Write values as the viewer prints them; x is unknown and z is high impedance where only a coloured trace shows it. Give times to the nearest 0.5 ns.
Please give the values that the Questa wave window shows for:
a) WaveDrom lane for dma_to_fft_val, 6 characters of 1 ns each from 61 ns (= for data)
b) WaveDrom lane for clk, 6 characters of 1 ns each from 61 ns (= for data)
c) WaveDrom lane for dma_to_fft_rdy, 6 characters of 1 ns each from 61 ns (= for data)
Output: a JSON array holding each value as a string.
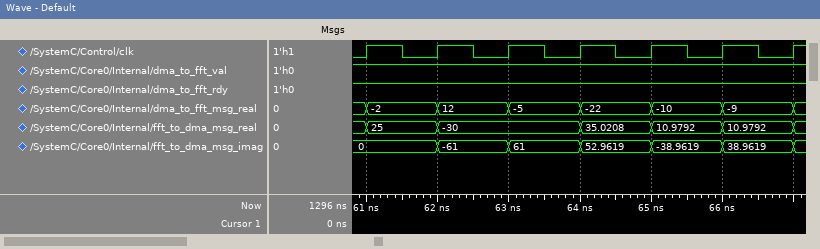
["{name: 'dma_to_fft_val', wave: '1.....'}", "{name: 'clk', wave: 'p.....'}", "{name: 'dma_to_fft_rdy', wave: '1.....'}"]
